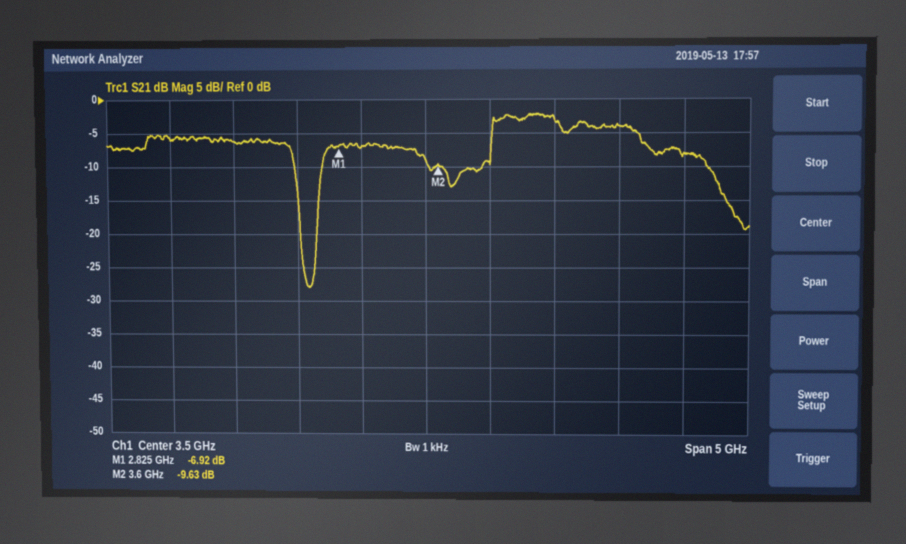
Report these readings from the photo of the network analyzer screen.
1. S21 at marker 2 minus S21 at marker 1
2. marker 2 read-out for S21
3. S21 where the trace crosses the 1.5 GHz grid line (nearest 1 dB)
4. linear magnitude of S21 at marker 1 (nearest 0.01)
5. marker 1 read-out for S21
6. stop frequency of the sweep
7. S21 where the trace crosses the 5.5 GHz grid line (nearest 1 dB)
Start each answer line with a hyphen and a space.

- -2.71 dB
- -9.63 dB
- -6 dB
- 0.45
- -6.92 dB
- 6 GHz
- -8 dB
